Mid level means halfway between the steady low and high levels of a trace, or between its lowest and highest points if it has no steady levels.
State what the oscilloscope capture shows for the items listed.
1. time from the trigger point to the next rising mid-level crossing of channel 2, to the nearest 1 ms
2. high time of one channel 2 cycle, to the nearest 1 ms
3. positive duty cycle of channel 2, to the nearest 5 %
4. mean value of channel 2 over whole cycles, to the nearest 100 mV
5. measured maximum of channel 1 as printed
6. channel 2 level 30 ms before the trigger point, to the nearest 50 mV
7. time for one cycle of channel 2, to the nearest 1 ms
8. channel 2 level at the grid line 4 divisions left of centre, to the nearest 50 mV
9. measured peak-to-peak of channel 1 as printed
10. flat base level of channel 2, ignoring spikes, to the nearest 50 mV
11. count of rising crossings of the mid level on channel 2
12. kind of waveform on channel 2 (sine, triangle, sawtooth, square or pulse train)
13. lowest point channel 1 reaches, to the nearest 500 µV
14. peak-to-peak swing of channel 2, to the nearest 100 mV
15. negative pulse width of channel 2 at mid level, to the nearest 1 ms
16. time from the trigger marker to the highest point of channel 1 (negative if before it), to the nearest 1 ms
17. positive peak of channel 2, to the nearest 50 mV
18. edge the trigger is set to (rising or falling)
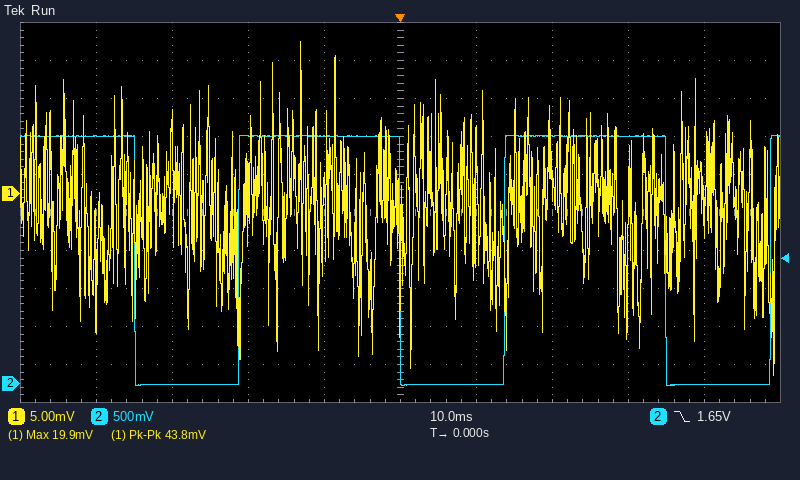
14 ms
21 ms
60 %
2.0 V
19.9 mV
0 mV
35 ms
3.25 V
43.8 mV
0 mV
3
pulse train
-24.0 mV
3.30 V
14 ms
-13 ms
3.25 V
falling
